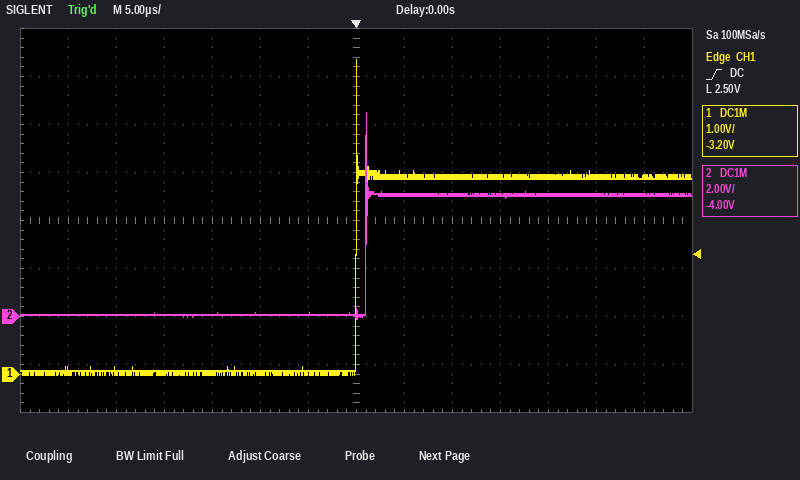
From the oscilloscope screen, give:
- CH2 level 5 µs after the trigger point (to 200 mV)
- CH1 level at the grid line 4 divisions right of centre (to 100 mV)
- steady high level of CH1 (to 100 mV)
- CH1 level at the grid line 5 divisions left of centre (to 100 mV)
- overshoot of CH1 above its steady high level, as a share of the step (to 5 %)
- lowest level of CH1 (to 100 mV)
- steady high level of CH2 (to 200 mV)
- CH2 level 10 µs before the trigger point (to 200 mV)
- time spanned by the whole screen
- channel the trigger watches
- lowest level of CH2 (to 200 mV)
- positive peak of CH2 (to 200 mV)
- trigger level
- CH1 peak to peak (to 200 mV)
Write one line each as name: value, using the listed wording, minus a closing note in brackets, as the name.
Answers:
CH2 level 5 µs after the trigger point: 5.0 V
CH1 level at the grid line 4 divisions right of centre: 4.1 V
steady high level of CH1: 4.1 V
CH1 level at the grid line 5 divisions left of centre: 100 mV
overshoot of CH1 above its steady high level, as a share of the step: 60 %
lowest level of CH1: 0.0 V
steady high level of CH2: 5.0 V
CH2 level 10 µs before the trigger point: 0.0 V
time spanned by the whole screen: 70 µs
channel the trigger watches: CH1
lowest level of CH2: 0.0 V
positive peak of CH2: 8.4 V
trigger level: 2.50 V
CH1 peak to peak: 6.6 V
